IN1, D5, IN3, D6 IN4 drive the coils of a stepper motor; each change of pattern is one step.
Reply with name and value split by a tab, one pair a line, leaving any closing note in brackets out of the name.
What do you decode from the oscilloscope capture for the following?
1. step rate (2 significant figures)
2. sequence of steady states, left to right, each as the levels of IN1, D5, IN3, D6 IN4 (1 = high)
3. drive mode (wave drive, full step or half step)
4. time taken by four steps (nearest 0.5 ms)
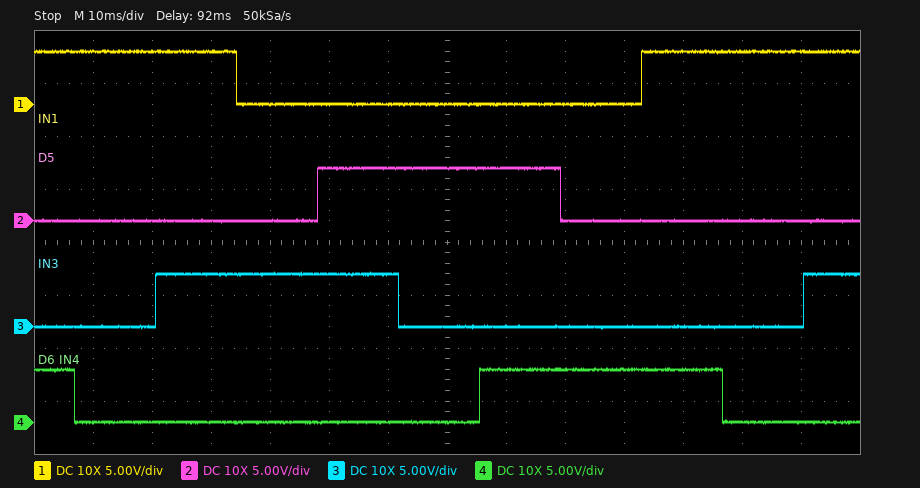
step rate	73 steps/s
sequence of steady states, left to right, each as the levels of IN1, D5, IN3, D6 IN4	1001 1000 1010 0010 0110 0100 0101 0001 1001 1000 1010
drive mode	half step
time taken by four steps	55.0 ms
